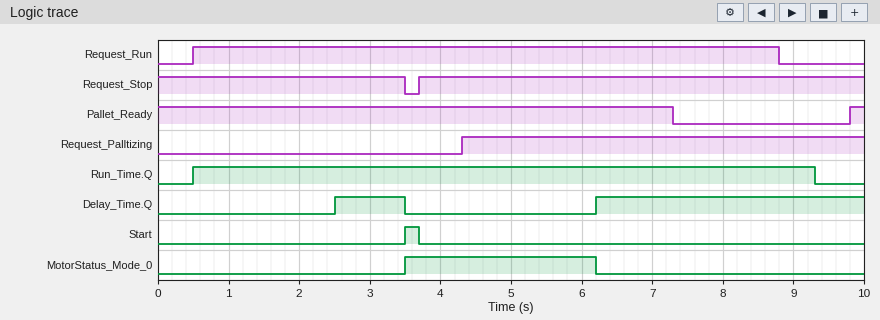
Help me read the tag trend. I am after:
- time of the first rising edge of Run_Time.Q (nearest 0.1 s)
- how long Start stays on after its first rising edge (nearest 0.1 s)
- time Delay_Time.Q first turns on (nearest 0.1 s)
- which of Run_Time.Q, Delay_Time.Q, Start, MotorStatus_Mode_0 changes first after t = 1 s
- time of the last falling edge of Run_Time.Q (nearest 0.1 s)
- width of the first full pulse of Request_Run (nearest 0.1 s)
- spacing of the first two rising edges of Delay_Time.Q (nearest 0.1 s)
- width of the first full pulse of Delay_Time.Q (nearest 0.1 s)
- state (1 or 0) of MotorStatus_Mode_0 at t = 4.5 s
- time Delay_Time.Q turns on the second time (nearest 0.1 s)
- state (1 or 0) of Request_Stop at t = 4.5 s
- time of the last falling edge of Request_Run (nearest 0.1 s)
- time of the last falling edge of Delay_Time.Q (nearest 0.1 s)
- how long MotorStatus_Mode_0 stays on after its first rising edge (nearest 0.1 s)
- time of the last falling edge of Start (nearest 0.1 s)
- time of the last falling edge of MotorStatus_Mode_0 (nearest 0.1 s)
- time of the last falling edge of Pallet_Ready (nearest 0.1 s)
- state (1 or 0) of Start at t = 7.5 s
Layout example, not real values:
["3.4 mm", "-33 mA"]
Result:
["0.5 s", "0.2 s", "2.5 s", "Delay_Time.Q", "9.3 s", "8.3 s", "3.7 s", "1.0 s", "1", "6.2 s", "1", "8.8 s", "3.5 s", "2.7 s", "3.7 s", "6.2 s", "7.3 s", "0"]
